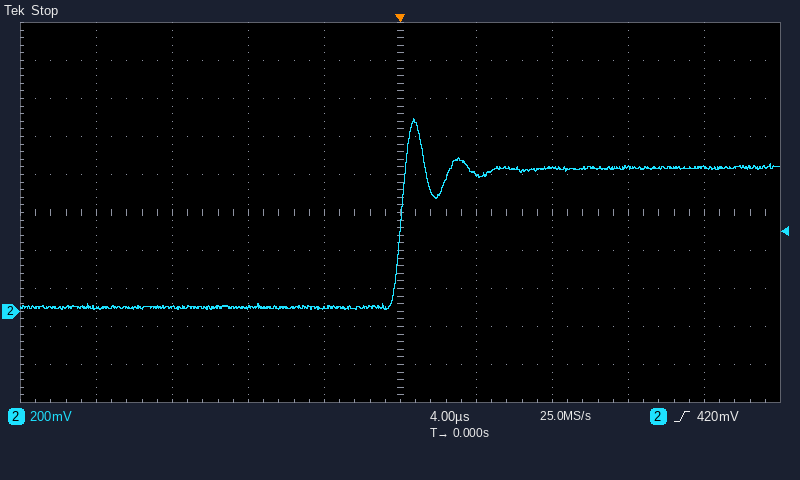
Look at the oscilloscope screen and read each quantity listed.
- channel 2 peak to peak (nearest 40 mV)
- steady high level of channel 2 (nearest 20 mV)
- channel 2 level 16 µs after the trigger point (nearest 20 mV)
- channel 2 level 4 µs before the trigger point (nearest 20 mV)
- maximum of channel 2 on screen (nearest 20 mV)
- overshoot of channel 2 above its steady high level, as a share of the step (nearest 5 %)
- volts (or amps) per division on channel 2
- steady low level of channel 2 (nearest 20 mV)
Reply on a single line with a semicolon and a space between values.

1.00 V; 760 mV; 760 mV; 20 mV; 1.02 V; 35 %; 200 mV; 20 mV
